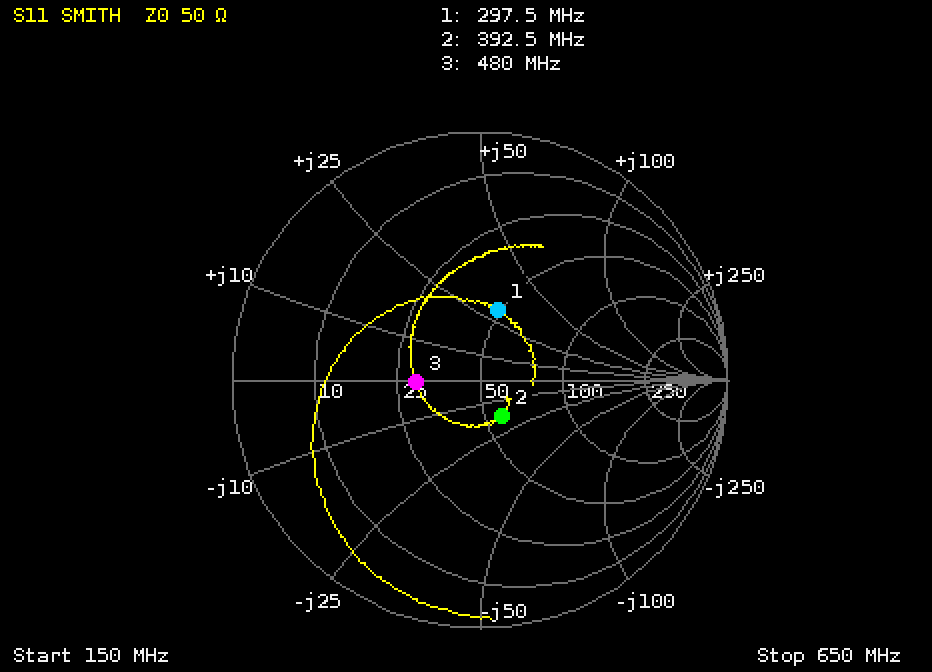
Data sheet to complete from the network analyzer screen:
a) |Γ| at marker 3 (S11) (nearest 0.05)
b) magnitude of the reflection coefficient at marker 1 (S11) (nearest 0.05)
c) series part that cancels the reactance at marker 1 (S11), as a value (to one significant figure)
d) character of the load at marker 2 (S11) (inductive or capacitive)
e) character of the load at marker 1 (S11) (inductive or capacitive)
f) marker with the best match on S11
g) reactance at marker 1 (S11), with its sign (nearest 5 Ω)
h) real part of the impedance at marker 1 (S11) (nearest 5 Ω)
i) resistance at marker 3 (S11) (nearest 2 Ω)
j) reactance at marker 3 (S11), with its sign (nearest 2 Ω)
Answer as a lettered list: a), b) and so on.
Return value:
a) 0.25
b) 0.30
c) 20 pF
d) capacitive
e) inductive
f) marker 2
g) +30 Ω
h) 50 Ω
i) 30 Ω
j) 0 Ω
